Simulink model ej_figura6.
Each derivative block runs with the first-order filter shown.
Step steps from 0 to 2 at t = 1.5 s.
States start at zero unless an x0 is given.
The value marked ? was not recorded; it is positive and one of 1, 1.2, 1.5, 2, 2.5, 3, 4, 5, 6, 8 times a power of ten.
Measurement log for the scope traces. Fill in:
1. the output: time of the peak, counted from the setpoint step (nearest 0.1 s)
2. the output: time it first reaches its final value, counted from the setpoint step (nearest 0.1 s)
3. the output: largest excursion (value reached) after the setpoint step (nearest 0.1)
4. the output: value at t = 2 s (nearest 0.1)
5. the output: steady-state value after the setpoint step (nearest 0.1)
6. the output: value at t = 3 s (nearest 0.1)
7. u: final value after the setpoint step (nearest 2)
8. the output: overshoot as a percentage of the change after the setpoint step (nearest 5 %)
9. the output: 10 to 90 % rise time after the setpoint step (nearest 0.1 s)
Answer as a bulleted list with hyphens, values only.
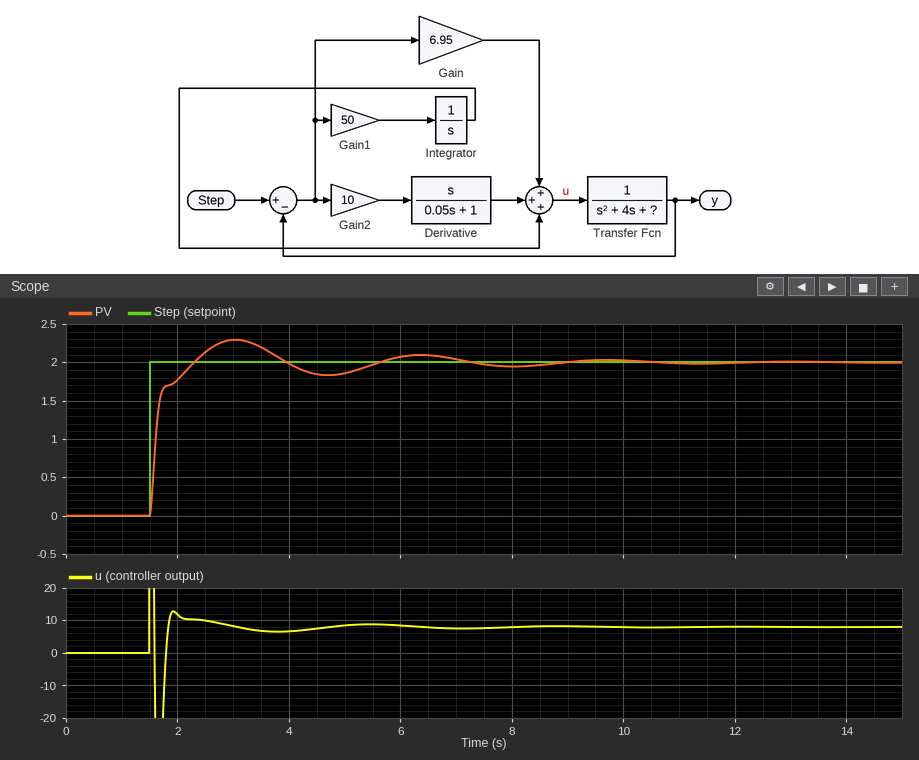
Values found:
- 1.5 s
- 0.8 s
- 2.3
- 1.8
- 2.0
- 2.3
- 8
- 15 %
- 0.5 s
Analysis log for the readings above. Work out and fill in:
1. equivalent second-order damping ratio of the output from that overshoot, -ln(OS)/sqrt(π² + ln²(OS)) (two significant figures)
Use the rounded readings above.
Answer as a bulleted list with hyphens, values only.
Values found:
- 0.52
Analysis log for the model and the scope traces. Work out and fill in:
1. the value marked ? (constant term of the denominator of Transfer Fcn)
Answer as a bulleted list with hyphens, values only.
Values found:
- 4
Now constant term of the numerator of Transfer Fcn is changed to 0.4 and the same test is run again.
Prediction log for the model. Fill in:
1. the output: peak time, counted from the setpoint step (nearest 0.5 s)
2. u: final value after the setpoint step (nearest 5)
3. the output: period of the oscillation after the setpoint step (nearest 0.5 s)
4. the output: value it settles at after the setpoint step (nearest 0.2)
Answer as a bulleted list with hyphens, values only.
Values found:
- 2.0 s
- 20
- 4.0 s
- 2.0
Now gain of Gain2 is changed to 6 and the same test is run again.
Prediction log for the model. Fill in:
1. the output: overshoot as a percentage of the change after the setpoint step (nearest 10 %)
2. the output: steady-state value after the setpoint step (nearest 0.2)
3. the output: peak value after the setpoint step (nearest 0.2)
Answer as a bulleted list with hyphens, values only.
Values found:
- 20 %
- 2.0
- 2.4
